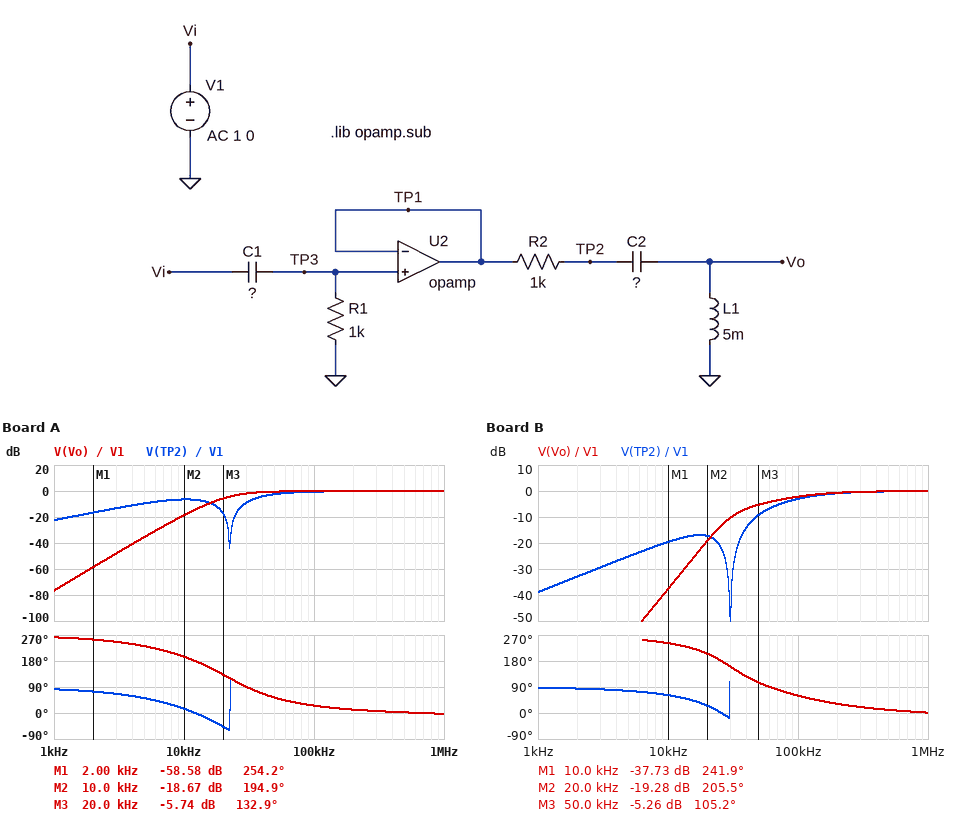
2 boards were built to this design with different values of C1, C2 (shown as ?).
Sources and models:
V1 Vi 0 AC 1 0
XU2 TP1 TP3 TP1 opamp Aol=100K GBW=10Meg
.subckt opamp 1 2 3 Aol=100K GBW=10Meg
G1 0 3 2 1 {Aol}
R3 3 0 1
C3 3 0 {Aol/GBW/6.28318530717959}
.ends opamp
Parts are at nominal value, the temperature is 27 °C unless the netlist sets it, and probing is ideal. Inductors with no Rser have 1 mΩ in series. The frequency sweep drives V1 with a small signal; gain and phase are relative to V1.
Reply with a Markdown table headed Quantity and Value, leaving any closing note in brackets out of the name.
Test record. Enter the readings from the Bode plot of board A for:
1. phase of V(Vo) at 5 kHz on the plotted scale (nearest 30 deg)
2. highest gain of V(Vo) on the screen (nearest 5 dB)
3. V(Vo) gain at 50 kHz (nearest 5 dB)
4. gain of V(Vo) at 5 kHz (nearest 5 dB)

| Quantity | Value |
|---|---|
| phase of V(Vo) at 5 kHz on the plotted scale | 240 deg |
| highest gain of V(Vo) on the screen | 0 dB |
| V(Vo) gain at 50 kHz | 0 dB |
| gain of V(Vo) at 5 kHz | -35 dB |
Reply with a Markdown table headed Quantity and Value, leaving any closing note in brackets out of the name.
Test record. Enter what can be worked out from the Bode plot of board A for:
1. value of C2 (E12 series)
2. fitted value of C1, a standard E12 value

| Quantity | Value |
|---|---|
| value of C2 | 10 nF |
| fitted value of C1, a standard E12 value | 12 nF |
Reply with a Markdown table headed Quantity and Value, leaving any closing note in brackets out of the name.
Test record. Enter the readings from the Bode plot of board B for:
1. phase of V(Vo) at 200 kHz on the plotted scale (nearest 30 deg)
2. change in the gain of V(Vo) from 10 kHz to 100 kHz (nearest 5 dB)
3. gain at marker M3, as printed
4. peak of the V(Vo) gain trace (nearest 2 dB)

| Quantity | Value |
|---|---|
| phase of V(Vo) at 200 kHz on the plotted scale | 30 deg |
| change in the gain of V(Vo) from 10 kHz to 100 kHz | 35 dB |
| gain at marker M3, as printed | -5.26 dB |
| peak of the V(Vo) gain trace | 0 dB |
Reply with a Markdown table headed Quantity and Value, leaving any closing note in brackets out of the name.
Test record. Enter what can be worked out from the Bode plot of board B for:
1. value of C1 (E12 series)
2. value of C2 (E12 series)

| Quantity | Value |
|---|---|
| value of C1 | 1.8 nF |
| value of C2 | 5.6 nF |
